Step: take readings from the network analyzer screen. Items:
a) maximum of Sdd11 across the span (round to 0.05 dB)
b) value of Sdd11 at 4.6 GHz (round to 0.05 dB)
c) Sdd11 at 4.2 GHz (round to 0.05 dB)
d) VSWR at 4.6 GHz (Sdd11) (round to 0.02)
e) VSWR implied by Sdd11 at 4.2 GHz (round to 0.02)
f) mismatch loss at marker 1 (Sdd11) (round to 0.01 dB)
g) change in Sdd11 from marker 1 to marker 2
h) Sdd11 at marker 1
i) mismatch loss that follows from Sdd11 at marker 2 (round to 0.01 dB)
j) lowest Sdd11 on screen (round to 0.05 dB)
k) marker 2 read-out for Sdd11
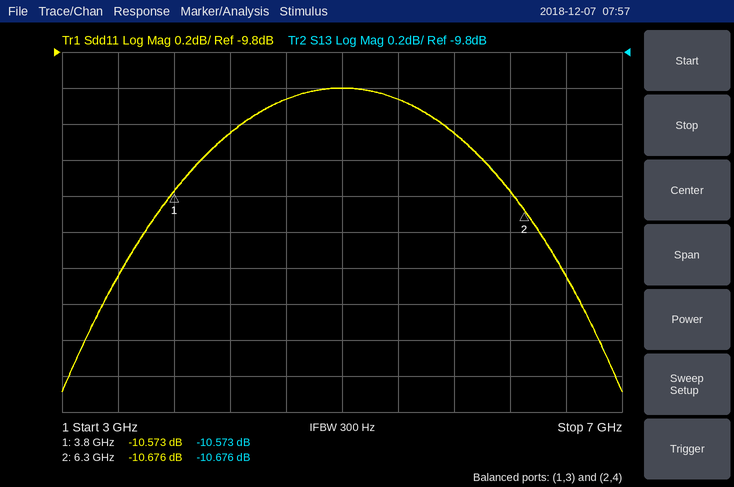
-10.00 dB
-10.05 dB
-10.25 dB
1.92
1.88
0.40 dB
-0.103 dB
-10.573 dB
0.39 dB
-11.70 dB
-10.676 dB
